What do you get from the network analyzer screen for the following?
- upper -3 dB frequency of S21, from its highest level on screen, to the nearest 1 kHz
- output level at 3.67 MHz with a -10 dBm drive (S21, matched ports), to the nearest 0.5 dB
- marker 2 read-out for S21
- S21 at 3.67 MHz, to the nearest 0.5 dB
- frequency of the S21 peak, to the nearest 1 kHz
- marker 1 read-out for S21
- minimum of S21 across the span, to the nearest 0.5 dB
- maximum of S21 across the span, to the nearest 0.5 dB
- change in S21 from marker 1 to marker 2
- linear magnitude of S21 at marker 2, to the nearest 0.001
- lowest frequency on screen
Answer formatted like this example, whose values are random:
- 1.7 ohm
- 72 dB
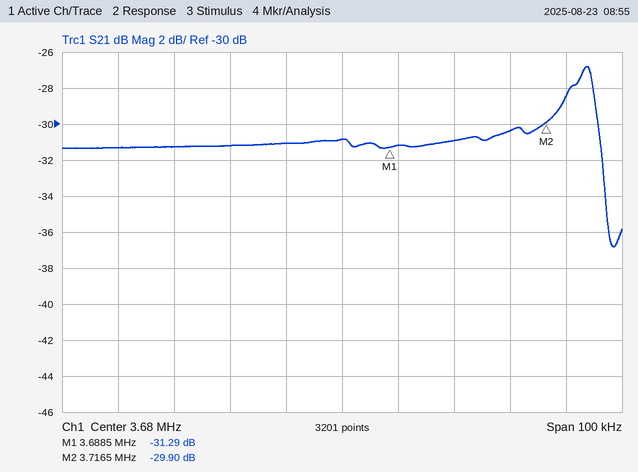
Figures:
- 3.726 MHz
- -41.0 dBm
- -29.90 dB
- -31.0 dB
- 3.724 MHz
- -31.29 dB
- -37.0 dB
- -27.0 dB
- 1.39 dB
- 0.032
- 3.63 MHz
